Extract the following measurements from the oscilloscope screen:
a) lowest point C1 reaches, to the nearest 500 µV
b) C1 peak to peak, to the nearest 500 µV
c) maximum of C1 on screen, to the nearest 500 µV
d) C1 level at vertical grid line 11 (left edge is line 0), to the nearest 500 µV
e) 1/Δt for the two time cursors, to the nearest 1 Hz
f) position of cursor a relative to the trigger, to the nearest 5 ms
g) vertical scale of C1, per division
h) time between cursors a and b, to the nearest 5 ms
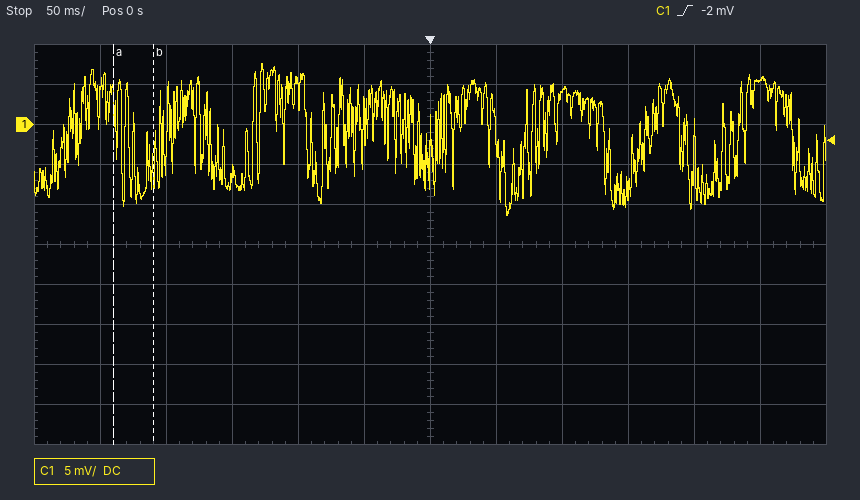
-11.5 mV
19.0 mV
7.5 mV
5.5 mV
33 Hz
-240 ms
5 mV
30 ms
